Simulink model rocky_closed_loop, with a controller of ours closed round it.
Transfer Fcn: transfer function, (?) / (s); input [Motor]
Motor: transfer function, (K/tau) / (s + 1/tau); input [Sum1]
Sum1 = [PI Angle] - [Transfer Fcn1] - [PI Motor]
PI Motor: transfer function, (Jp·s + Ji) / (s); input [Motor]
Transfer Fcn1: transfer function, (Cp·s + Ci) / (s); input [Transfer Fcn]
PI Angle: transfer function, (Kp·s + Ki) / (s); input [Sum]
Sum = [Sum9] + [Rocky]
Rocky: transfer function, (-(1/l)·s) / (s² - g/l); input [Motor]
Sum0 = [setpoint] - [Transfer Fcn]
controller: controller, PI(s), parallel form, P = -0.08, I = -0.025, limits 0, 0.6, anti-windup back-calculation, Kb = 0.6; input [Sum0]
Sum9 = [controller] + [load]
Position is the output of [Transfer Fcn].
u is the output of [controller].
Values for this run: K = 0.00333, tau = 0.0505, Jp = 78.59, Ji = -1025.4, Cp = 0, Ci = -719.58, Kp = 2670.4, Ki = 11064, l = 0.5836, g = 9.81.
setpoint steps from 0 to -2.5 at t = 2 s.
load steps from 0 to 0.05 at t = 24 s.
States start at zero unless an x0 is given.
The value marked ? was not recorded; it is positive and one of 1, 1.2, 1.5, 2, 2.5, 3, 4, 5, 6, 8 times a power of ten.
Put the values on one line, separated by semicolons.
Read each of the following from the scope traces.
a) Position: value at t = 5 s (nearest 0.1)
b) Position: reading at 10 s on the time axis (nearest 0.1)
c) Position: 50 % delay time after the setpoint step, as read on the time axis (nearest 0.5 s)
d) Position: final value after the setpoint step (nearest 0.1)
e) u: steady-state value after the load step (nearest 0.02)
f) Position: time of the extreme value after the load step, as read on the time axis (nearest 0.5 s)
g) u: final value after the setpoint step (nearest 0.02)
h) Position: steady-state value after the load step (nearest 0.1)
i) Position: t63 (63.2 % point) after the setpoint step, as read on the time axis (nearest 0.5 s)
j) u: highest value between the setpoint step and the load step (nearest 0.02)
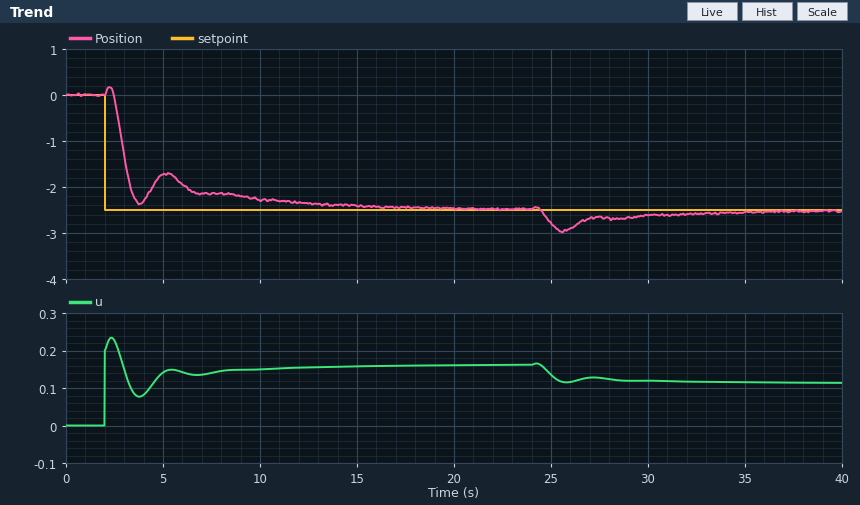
-1.7; -2.3; 3.0 s; -2.5; 0.12; 25.5 s; 0.16; -2.5; 3.0 s; 0.24
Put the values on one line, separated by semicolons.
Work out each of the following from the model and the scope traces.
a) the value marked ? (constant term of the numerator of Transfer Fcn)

1
